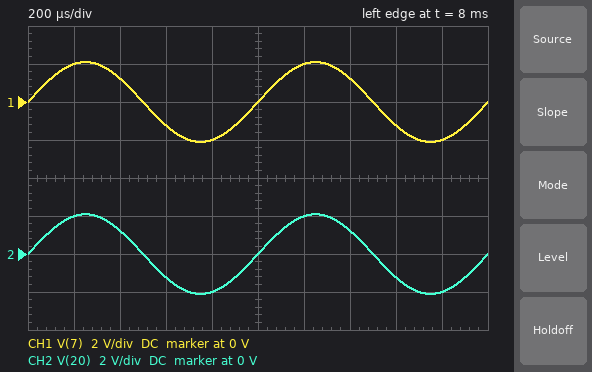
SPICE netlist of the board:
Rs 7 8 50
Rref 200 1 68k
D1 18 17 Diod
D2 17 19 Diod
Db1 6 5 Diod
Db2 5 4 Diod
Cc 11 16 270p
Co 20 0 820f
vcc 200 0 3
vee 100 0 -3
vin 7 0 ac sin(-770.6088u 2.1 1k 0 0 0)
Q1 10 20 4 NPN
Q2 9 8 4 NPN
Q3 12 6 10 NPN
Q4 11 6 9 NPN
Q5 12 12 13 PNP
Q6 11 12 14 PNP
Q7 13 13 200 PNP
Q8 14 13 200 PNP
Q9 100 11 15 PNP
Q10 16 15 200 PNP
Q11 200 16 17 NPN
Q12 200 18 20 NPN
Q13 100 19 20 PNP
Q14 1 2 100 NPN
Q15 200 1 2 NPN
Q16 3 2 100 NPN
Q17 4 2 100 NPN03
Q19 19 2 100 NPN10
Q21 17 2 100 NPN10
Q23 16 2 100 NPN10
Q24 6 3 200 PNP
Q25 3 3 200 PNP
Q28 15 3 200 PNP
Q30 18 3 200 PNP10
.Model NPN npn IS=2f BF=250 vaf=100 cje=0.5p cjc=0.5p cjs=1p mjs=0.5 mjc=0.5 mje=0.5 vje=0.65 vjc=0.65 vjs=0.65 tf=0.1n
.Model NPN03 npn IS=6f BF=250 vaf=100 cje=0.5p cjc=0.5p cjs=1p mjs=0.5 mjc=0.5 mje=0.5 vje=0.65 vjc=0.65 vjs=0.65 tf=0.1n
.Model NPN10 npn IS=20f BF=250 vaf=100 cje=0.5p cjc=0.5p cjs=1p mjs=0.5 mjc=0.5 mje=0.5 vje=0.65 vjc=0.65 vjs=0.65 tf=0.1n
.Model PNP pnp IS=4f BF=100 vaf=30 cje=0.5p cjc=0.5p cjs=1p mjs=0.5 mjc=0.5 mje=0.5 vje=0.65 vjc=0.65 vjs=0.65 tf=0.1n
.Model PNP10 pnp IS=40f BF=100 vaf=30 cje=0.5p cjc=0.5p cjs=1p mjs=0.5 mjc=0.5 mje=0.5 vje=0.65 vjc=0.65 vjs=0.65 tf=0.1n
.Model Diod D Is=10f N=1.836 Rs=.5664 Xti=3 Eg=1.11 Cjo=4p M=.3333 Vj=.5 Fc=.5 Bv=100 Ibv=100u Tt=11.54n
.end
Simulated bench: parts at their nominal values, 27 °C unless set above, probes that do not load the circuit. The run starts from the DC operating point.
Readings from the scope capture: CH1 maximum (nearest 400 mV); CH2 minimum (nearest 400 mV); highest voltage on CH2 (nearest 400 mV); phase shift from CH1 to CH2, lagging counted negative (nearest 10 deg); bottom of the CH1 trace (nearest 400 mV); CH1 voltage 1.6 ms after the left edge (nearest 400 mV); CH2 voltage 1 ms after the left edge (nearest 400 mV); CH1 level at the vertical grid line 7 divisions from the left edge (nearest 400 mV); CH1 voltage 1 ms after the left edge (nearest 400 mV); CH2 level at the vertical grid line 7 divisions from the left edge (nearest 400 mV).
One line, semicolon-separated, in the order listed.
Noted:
2.0 V; -2.0 V; 2.0 V; 0 deg; -2.0 V; -1.2 V; 0 V; 1.2 V; 0 V; 1.2 V
